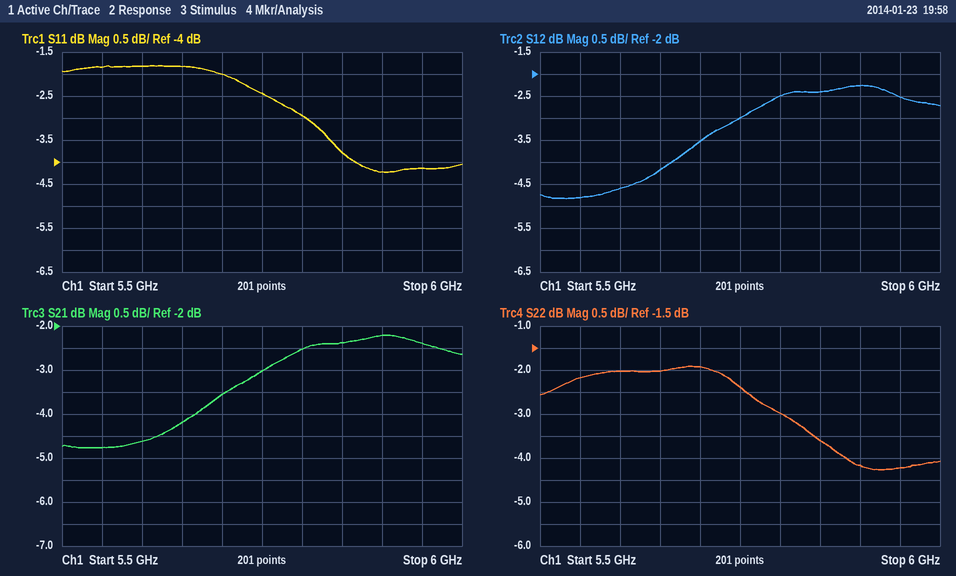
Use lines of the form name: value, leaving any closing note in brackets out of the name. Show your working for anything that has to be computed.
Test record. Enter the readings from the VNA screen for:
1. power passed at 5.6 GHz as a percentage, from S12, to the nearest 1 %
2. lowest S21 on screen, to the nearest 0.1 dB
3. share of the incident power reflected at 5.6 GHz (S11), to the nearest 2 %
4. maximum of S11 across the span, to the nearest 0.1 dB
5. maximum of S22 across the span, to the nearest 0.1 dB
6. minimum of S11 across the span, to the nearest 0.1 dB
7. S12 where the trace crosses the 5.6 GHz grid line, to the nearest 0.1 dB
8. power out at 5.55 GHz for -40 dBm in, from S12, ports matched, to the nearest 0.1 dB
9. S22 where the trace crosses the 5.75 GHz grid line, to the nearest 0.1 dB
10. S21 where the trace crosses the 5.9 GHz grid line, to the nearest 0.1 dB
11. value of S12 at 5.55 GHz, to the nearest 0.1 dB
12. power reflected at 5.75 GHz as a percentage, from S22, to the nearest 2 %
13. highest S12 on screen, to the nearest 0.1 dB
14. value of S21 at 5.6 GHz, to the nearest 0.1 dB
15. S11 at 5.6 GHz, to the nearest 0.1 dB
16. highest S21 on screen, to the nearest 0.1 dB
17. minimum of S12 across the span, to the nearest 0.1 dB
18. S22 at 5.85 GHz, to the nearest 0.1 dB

power passed at 5.6 GHz as a percentage, from S12, to the nearest 1 %: 10^(-4.6/10) ≈ 35 %
lowest S21 on screen, to the nearest 0.1 dB: -4.8 dB
share of the incident power reflected at 5.6 GHz (S11), to the nearest 2 %: 10^(-1.8/10) ≈ 66 %
maximum of S11 across the span, to the nearest 0.1 dB: -1.8 dB
maximum of S22 across the span, to the nearest 0.1 dB: -1.9 dB
minimum of S11 across the span, to the nearest 0.1 dB: -4.2 dB
S12 where the trace crosses the 5.6 GHz grid line, to the nearest 0.1 dB: -4.6 dB
power out at 5.55 GHz for -40 dBm in, from S12, ports matched, to the nearest 0.1 dB: -40 dBm + (-4.8 dB) = -44.8 dBm
S22 where the trace crosses the 5.75 GHz grid line, to the nearest 0.1 dB: -2.4 dB
S21 where the trace crosses the 5.9 GHz grid line, to the nearest 0.1 dB: -2.2 dB
value of S12 at 5.55 GHz, to the nearest 0.1 dB: -4.8 dB
power reflected at 5.75 GHz as a percentage, from S22, to the nearest 2 %: 10^(-2.4/10) ≈ 58 %
highest S12 on screen, to the nearest 0.1 dB: -2.3 dB
value of S21 at 5.6 GHz, to the nearest 0.1 dB: -4.6 dB
S11 at 5.6 GHz, to the nearest 0.1 dB: -1.8 dB
highest S21 on screen, to the nearest 0.1 dB: -2.2 dB
minimum of S12 across the span, to the nearest 0.1 dB: -4.8 dB
S22 at 5.85 GHz, to the nearest 0.1 dB: -3.6 dB
